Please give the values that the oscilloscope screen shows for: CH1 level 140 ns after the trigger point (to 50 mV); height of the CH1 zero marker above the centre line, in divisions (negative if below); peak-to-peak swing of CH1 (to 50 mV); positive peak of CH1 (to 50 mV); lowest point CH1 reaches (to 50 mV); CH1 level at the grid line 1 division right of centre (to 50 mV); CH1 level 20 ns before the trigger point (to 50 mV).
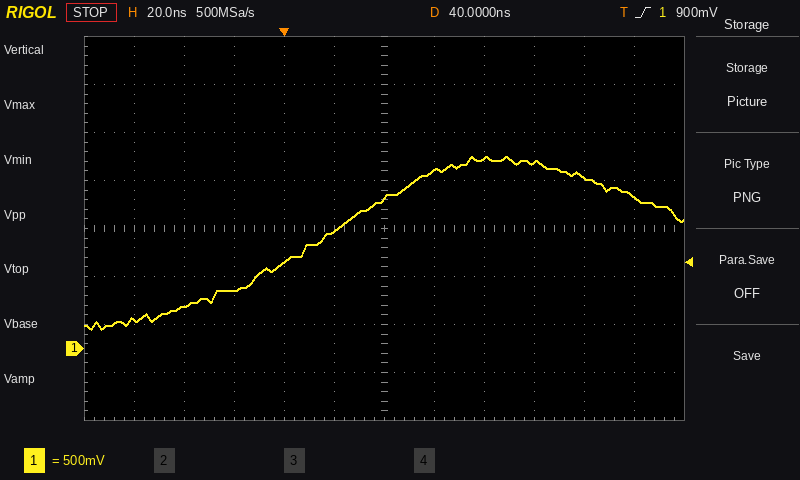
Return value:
1.60 V
-2.5 div
1.80 V
2.00 V
200 mV
1.85 V
600 mV
